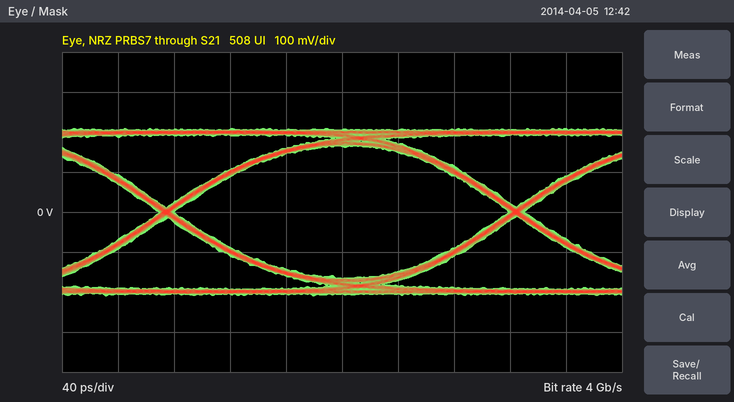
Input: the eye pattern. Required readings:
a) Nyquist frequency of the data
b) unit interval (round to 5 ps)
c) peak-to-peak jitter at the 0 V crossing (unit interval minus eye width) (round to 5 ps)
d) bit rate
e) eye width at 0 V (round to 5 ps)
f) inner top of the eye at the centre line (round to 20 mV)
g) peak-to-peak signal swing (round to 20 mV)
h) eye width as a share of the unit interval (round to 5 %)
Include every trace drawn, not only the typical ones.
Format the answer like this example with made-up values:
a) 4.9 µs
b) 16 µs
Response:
a) 2 GHz
b) 250 ps
c) 10 ps
d) 4 Gb/s
e) 240 ps
f) 160 mV
g) 420 mV
h) 95 %
